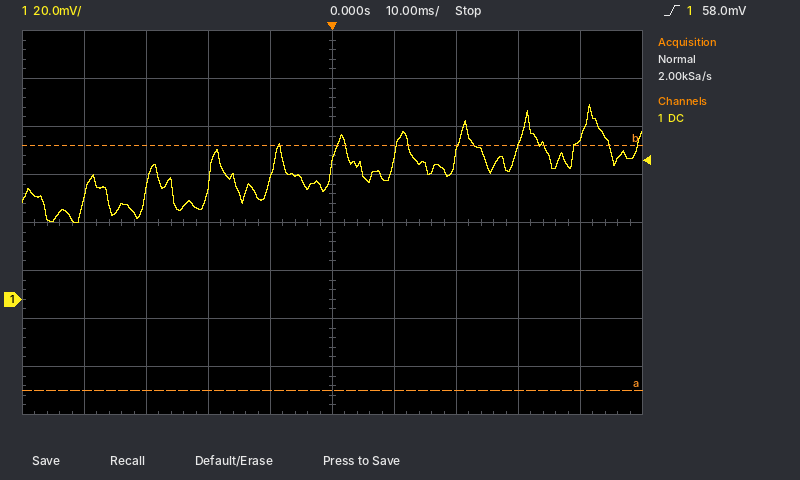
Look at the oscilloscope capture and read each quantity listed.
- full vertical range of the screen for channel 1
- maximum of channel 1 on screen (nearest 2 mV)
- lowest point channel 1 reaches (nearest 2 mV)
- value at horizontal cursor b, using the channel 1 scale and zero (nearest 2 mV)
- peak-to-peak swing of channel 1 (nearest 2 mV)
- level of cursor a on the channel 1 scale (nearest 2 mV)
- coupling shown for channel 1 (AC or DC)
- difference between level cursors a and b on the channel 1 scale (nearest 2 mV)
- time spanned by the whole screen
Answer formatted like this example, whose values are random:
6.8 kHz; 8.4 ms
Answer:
160 mV; 82 mV; 32 mV; 64 mV; 50 mV; -38 mV; DC; 102 mV; 100 ms
